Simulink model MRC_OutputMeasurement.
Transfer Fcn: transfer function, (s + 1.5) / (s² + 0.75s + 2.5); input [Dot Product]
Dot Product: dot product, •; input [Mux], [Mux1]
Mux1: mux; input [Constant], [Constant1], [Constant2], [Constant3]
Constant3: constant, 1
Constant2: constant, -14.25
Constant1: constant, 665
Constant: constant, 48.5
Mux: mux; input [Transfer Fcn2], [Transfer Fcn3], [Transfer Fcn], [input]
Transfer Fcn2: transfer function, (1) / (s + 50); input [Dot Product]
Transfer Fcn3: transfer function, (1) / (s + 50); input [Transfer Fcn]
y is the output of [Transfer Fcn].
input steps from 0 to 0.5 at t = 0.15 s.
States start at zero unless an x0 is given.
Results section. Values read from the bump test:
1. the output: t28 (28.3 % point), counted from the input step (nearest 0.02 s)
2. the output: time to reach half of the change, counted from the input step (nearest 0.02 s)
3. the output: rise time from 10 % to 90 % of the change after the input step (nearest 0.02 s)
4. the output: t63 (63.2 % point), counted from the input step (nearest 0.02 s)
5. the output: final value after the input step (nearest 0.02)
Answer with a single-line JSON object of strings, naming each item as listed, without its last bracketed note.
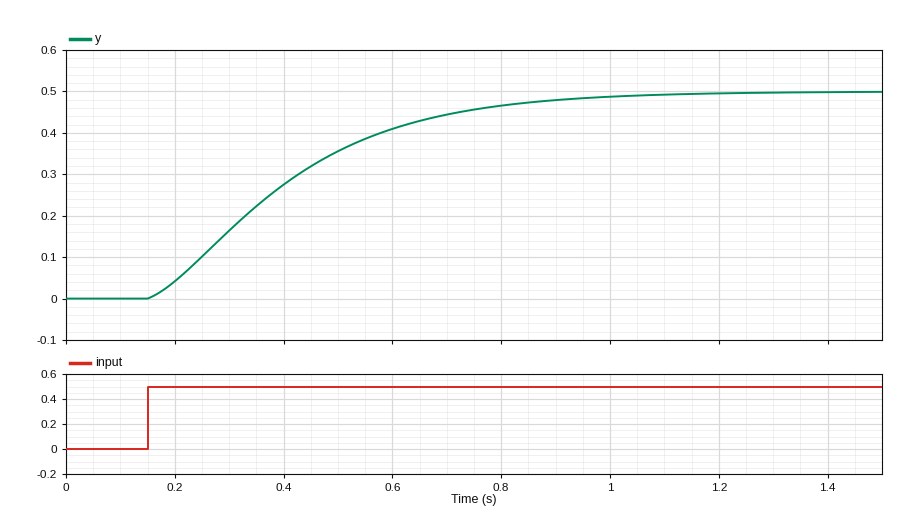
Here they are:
{"the output: t28 (28.3 % point), counted from the input step": "0.14 s", "the output: time to reach half of the change, counted from the input step": "0.22 s", "the output: rise time from 10 % to 90 % of the change after the input step": "0.52 s", "the output: t63 (63.2 % point), counted from the input step": "0.30 s", "the output: final value after the input step": "0.50"}
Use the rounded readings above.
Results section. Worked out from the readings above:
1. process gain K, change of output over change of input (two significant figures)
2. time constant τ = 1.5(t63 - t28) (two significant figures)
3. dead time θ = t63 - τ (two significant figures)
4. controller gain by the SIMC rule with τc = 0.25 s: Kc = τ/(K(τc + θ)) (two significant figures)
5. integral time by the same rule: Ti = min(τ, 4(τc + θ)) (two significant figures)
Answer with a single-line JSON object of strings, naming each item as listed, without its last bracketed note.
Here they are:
{"process gain K, change of output over change of input": "1.0", "time constant τ = 1.5(t63 - t28)": "0.24 s", "dead time θ = t63 - τ": "0.060 s", "controller gain by the SIMC rule with τc = 0.25 s: Kc = τ/(K(τc + θ))": "0.77", "integral time by the same rule: Ti = min(τ, 4(τc + θ))": "0.24 s"}
